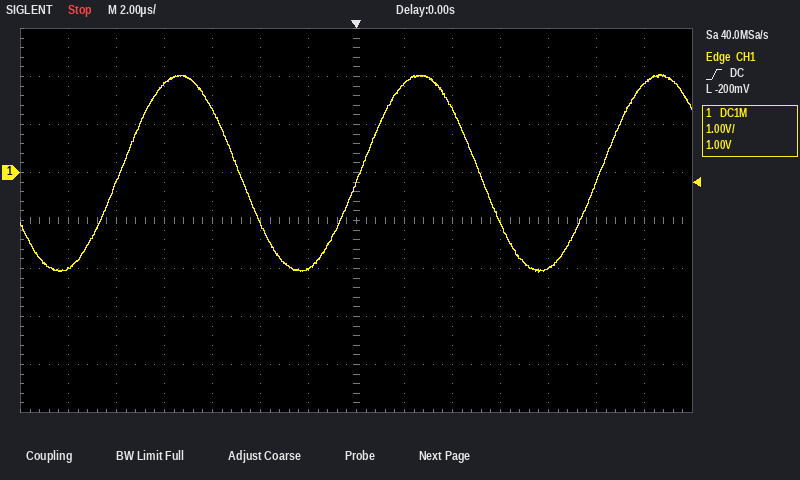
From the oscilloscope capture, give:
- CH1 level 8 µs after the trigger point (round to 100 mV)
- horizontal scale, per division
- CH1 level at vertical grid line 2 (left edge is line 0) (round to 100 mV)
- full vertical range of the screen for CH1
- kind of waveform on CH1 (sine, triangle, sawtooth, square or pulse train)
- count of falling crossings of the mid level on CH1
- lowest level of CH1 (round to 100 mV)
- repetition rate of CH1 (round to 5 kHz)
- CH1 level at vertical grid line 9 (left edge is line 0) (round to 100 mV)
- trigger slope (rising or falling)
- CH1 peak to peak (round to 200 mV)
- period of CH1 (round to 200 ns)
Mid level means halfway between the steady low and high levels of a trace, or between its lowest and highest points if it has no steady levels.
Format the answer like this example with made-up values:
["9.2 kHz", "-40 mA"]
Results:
["-2.0 V", "2 µs", "-200 mV", "8 V", "sine", "2", "-2.1 V", "100 kHz", "1.3 V", "rising", "4.2 V", "10.0 µs"]
